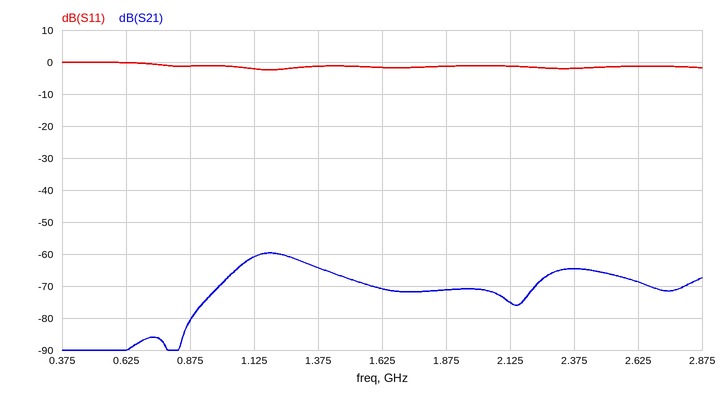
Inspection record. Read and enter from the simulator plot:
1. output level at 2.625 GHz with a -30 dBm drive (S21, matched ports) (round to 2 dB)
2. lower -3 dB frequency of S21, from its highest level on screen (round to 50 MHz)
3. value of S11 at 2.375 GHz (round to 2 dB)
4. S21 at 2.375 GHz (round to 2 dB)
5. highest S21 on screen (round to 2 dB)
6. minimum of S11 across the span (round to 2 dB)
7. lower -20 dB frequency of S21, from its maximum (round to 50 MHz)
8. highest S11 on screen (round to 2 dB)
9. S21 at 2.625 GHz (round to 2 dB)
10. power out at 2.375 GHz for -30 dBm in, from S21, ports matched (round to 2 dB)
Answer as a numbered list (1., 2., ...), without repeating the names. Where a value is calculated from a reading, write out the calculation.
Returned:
1. -30 dBm + (-68 dB) = -98 dBm
2. 1.10 GHz
3. -2 dB
4. -64 dB
5. -60 dB
6. -2 dB
7. 900 MHz
8. 0 dB
9. -68 dB
10. -30 dBm + (-64 dB) = -94 dBm
